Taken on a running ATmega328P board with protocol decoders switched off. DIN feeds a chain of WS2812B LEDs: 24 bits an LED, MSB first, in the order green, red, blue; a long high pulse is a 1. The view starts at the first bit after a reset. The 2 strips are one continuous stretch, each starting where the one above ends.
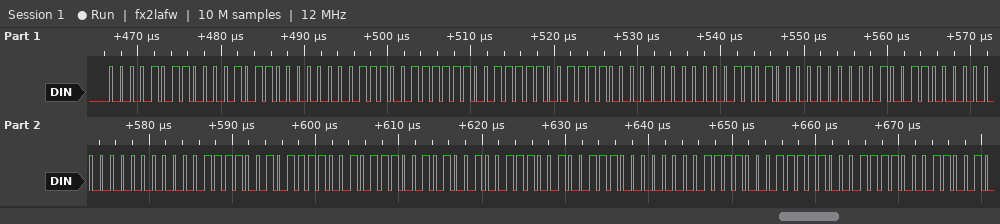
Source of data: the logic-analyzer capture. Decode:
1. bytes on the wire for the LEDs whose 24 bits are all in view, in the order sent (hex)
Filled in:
0B 0B 00 E7 E7 CF 00 0D 00 26 00 00 F2 F2 E5 27 27 00 F1 F1 E3
